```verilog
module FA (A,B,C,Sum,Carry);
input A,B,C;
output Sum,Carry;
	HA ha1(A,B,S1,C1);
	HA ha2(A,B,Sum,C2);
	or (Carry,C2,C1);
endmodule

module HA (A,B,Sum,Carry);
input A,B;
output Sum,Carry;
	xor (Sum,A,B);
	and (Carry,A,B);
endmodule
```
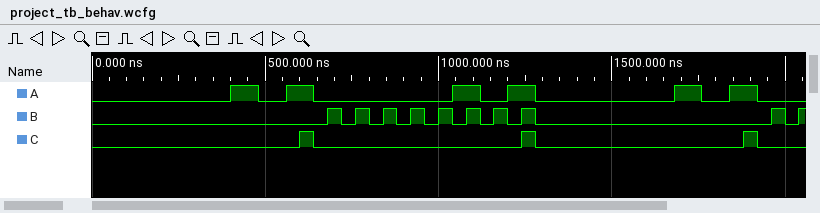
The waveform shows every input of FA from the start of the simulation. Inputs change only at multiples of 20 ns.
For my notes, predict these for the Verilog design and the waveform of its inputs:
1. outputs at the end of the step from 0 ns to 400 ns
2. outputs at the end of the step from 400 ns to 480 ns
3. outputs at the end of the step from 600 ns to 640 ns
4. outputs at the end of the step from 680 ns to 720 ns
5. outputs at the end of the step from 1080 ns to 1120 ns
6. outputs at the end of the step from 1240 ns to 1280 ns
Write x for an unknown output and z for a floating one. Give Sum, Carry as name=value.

Sum=0, Carry=0
Sum=1, Carry=0
Sum=1, Carry=0
Sum=1, Carry=0
Sum=0, Carry=1
Sum=0, Carry=1
